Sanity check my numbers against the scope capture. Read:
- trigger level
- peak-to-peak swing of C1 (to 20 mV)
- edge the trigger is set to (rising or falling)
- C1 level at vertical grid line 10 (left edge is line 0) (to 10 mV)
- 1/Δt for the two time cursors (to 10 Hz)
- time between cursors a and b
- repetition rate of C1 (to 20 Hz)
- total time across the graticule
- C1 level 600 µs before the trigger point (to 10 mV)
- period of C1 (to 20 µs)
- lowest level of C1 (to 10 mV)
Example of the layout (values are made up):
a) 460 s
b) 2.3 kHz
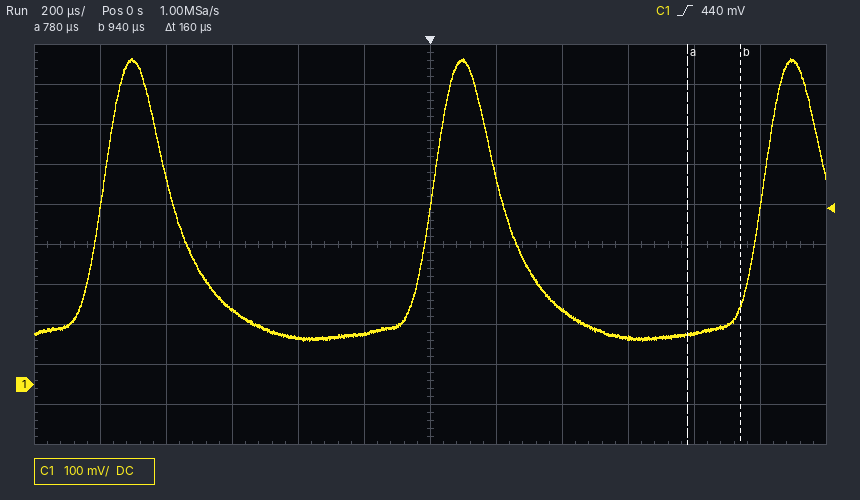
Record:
a) 440 mV
b) 700 mV
c) rising
d) 130 mV
e) 6.25 kHz
f) 160 µs
g) 1.00 kHz
h) 2.4 ms
i) 190 mV
j) 1.00 ms
k) 110 mV
